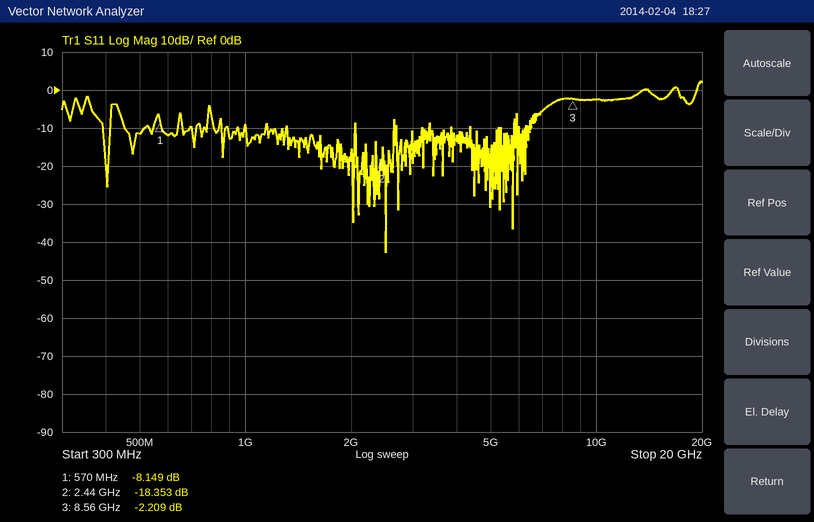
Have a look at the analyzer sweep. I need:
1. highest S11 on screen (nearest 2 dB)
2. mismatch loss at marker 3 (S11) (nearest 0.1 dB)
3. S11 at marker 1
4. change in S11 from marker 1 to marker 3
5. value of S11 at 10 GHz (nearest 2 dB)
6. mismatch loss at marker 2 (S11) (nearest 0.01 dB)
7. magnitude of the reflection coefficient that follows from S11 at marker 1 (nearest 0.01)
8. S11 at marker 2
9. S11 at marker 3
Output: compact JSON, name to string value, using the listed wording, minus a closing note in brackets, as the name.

{"highest S11 on screen": "2 dB", "mismatch loss at marker 3 (S11)": "4.0 dB", "S11 at marker 1": "-8.149 dB", "change in S11 from marker 1 to marker 3": "5.940 dB", "value of S11 at 10 GHz": "-2 dB", "mismatch loss at marker 2 (S11)": "0.06 dB", "magnitude of the reflection coefficient that follows from S11 at marker 1": "0.39", "S11 at marker 2": "-18.353 dB", "S11 at marker 3": "-2.209 dB"}
